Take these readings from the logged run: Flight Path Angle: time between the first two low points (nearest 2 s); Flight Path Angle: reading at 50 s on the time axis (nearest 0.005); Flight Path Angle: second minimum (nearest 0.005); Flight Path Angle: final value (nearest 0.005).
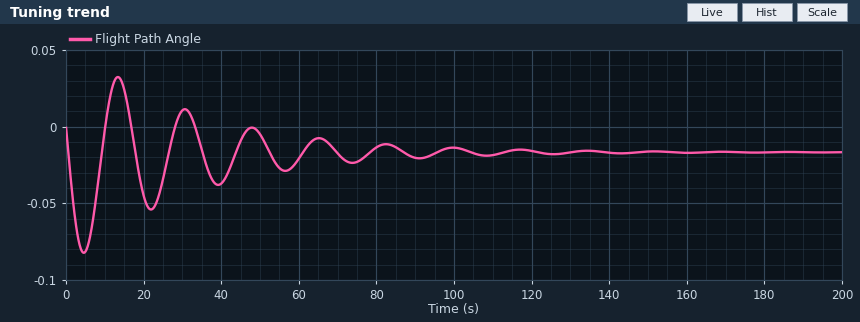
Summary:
18 s
-0.005
-0.055
-0.015
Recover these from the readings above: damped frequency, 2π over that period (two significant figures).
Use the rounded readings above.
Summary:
0.35 rad/s
